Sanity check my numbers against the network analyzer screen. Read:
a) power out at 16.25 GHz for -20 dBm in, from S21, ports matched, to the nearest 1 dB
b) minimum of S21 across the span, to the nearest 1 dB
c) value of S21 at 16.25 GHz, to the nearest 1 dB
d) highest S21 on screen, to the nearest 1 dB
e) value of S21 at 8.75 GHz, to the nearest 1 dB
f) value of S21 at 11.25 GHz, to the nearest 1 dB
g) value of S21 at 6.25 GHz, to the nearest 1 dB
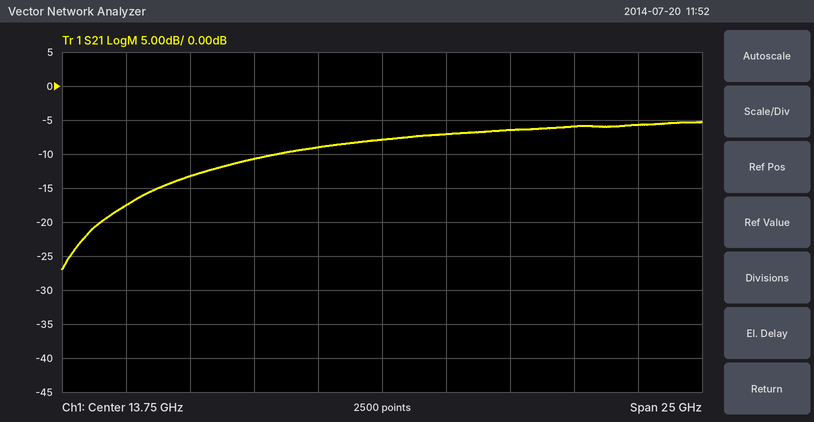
-27 dBm
-27 dB
-7 dB
-5 dB
-11 dB
-9 dB
-13 dB
